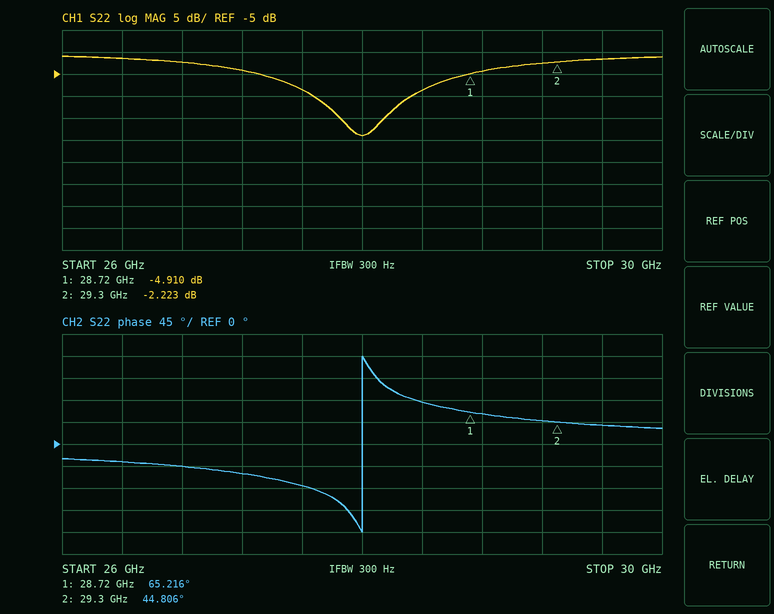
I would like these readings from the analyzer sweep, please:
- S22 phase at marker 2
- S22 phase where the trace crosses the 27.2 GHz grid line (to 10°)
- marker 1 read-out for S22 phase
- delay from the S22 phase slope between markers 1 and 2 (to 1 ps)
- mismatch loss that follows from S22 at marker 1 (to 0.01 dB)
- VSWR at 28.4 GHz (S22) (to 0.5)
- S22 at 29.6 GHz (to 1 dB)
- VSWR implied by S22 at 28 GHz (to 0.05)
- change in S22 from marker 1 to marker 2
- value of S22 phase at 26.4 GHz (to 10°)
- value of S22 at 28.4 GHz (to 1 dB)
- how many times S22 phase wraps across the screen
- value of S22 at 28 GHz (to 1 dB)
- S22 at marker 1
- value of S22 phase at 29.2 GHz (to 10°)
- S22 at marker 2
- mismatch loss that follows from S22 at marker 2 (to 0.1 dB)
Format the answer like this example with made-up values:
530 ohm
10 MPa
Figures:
44.806°
-60°
65.216°
98 ps
1.69 dB
2.0
-2 dB
1.25
2.687 dB
-40°
-9 dB
1
-19 dB
-4.910 dB
50°
-2.223 dB
4.0 dB
